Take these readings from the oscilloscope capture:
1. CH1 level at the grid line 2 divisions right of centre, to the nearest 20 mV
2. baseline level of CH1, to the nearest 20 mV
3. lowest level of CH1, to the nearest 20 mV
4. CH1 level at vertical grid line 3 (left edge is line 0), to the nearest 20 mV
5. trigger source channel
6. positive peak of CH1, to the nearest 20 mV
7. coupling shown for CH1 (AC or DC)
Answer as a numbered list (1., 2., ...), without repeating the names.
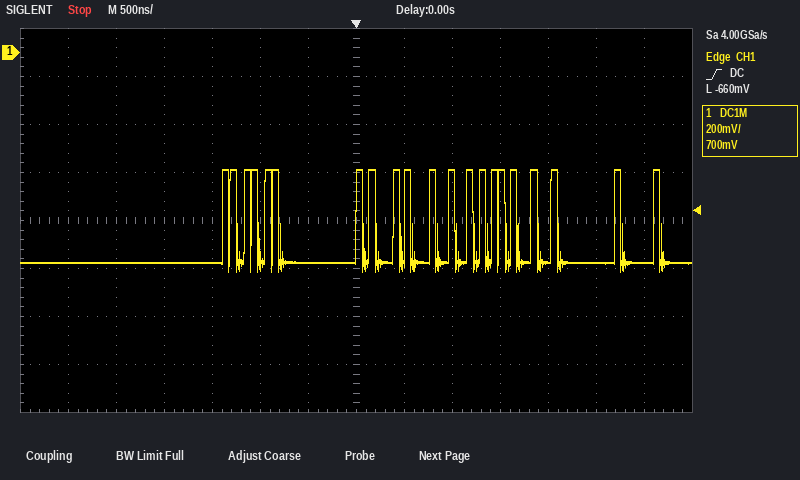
1. -480 mV
2. -880 mV
3. -920 mV
4. -880 mV
5. CH1
6. -480 mV
7. DC
